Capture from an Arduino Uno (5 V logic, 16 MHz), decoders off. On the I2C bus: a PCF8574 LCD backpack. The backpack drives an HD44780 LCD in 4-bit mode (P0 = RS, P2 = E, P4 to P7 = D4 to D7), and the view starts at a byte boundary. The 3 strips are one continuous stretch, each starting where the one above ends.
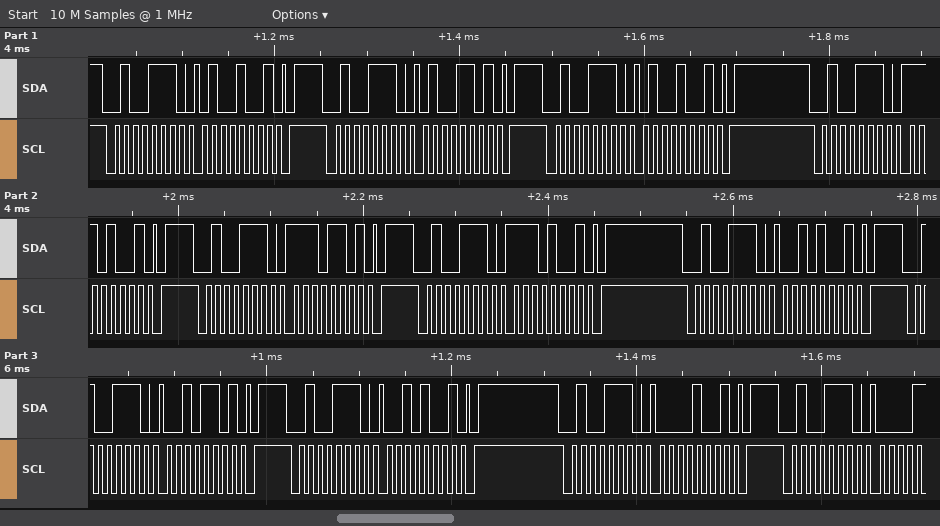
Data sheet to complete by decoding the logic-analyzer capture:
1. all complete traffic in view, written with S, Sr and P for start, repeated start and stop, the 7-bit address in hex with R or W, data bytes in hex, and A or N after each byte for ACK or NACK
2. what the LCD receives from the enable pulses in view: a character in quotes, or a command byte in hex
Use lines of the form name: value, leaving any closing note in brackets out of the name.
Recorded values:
all complete traffic in view, written with S, Sr and P for start, repeated start and stop, the 7-bit address in hex with R or W, data bytes in hex, and A or N after each byte for ACK or NACK: S 27W A 49 A P S 27W A 4D A P S 27W A 49 A P S 27W A E9 A P S 27W A ED A P S 27W A E9 A P S 27W A 29 A P S 27W A 2D A P S 27W A 29 A P S 27W A 09 A P S 27W A
what the LCD receives from the enable pulses in view: a character in quotes, or a command byte in hex: 'N'
